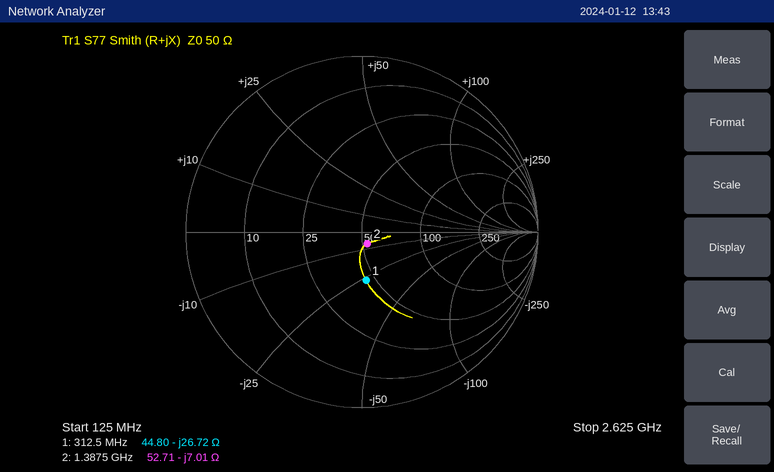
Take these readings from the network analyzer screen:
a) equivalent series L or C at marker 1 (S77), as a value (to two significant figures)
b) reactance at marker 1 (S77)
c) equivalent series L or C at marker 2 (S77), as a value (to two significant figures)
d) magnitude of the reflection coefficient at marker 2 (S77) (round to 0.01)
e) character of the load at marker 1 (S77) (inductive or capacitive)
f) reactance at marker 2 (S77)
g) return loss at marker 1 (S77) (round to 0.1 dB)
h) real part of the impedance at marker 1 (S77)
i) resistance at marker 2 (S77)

19 pF
-26.72 Ω
16 pF
0.07
capacitive
-7.01 Ω
11.2 dB
44.80 Ω
52.71 Ω
